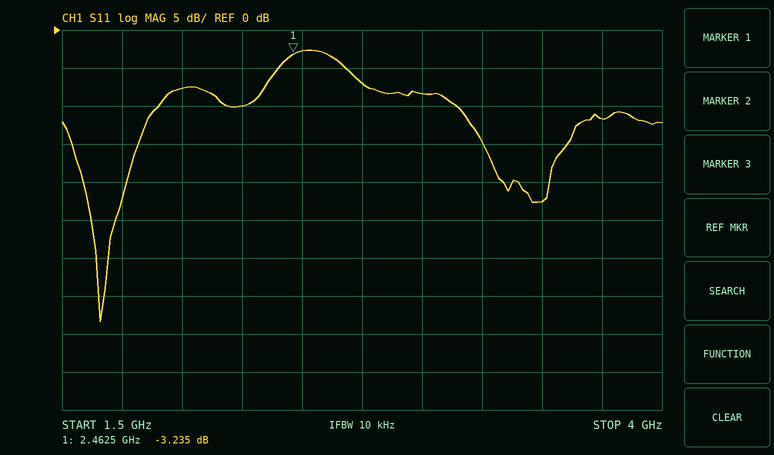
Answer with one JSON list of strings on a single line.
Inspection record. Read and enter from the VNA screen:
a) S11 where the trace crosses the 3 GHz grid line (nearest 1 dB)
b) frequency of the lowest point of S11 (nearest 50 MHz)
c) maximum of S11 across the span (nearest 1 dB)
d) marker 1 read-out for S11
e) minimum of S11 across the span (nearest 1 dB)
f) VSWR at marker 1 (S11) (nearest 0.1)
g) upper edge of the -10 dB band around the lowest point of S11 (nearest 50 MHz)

["-8 dB", "1.65 GHz", "-3 dB", "-3.235 dB", "-38 dB", "5.4", "1.90 GHz"]
